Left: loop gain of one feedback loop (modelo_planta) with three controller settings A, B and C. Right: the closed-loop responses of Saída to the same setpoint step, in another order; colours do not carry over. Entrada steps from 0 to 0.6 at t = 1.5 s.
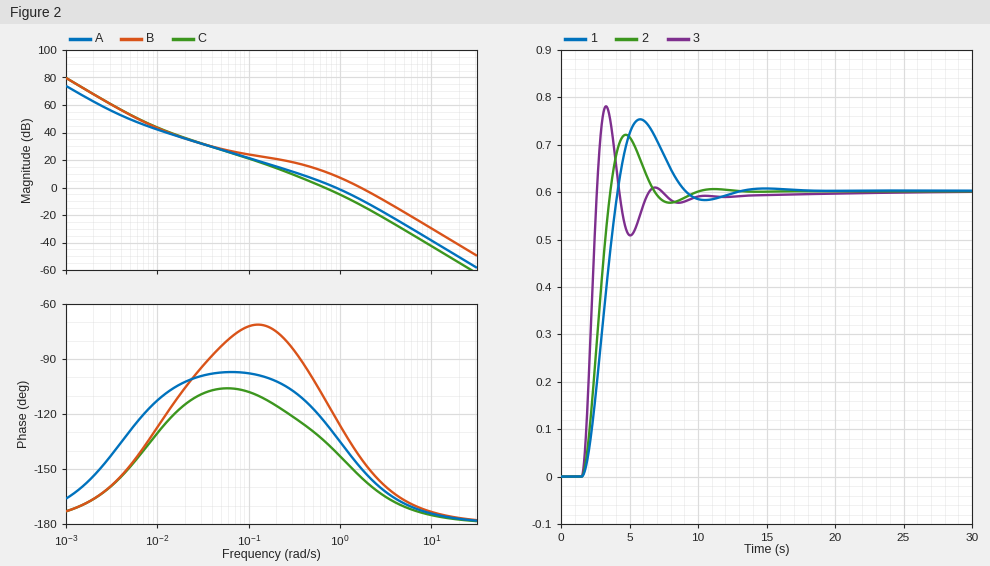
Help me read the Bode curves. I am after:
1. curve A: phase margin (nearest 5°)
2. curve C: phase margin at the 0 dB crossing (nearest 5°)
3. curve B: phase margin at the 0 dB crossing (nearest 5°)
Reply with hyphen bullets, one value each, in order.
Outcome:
- 50°
- 45°
- 35°
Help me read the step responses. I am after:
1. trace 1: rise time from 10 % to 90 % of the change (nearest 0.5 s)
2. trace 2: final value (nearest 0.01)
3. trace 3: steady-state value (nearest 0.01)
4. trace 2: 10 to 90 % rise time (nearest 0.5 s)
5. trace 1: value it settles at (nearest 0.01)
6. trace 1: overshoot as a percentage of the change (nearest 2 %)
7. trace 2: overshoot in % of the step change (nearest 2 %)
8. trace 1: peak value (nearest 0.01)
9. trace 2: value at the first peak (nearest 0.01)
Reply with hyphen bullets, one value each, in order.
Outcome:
- 2.0 s
- 0.60
- 0.60
- 1.5 s
- 0.60
- 26 %
- 20 %
- 0.75
- 0.72
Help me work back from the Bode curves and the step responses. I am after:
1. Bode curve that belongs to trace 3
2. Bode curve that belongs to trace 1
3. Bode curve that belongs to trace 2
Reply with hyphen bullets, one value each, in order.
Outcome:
- B
- C
- A
